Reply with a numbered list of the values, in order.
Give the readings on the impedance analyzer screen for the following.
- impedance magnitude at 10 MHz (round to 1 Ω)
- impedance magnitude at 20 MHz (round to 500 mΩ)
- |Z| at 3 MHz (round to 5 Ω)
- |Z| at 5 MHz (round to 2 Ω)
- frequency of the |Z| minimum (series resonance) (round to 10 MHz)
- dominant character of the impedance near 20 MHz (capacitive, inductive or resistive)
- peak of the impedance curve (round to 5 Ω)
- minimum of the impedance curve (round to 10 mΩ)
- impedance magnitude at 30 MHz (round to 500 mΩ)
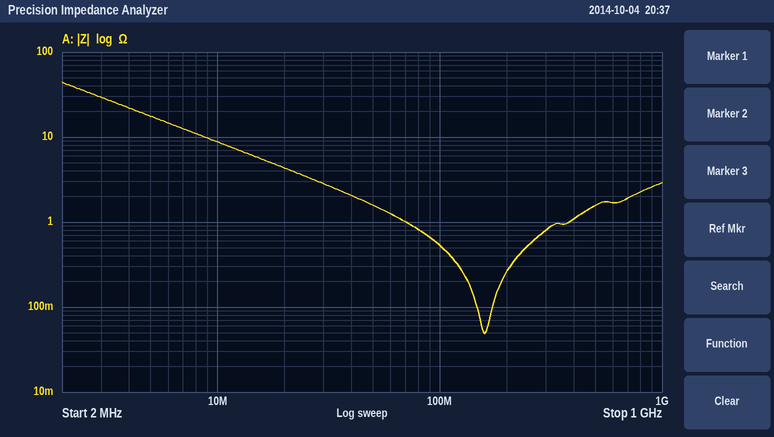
1. 9 Ω
2. 4.5 Ω
3. 30 Ω
4. 18 Ω
5. 160 MHz
6. capacitive
7. 45 Ω
8. 50 mΩ
9. 3.0 Ω
